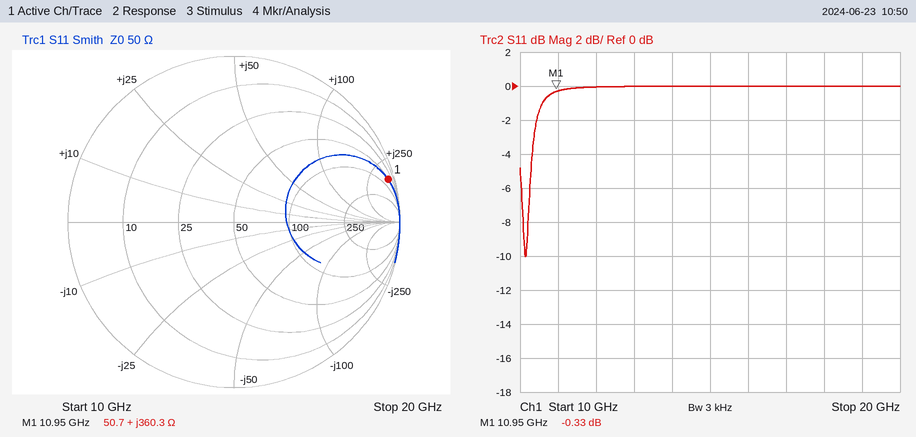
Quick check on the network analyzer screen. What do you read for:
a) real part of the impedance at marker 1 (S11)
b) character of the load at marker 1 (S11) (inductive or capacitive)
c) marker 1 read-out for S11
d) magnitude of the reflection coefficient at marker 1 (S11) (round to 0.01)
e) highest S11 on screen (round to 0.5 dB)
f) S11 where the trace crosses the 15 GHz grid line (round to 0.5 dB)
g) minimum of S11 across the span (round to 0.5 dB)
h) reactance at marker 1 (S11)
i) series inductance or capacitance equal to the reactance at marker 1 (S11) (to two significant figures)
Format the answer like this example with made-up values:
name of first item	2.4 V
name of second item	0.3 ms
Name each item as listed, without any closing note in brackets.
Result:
real part of the impedance at marker 1	50.7 Ω
character of the load at marker 1 (S11)	inductive
marker 1 read-out for S11	-0.33 dB
magnitude of the reflection coefficient at marker 1 (S11)	0.96
highest S11 on screen	0.0 dB
S11 where the trace crosses the 15 GHz grid line	0.0 dB
minimum of S11 across the span	-10.0 dB
reactance at marker 1	+360.3 Ω
series inductance or capacitance equal to the reactance at marker 1 (S11)	5.2 nH
